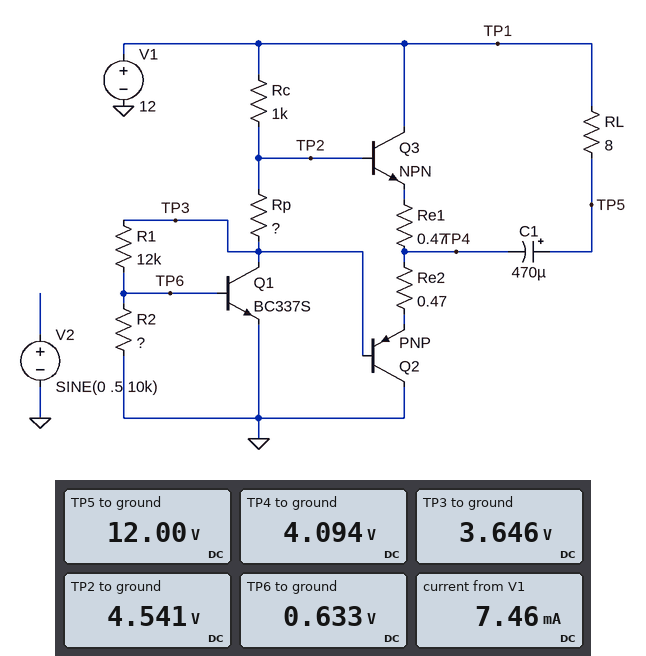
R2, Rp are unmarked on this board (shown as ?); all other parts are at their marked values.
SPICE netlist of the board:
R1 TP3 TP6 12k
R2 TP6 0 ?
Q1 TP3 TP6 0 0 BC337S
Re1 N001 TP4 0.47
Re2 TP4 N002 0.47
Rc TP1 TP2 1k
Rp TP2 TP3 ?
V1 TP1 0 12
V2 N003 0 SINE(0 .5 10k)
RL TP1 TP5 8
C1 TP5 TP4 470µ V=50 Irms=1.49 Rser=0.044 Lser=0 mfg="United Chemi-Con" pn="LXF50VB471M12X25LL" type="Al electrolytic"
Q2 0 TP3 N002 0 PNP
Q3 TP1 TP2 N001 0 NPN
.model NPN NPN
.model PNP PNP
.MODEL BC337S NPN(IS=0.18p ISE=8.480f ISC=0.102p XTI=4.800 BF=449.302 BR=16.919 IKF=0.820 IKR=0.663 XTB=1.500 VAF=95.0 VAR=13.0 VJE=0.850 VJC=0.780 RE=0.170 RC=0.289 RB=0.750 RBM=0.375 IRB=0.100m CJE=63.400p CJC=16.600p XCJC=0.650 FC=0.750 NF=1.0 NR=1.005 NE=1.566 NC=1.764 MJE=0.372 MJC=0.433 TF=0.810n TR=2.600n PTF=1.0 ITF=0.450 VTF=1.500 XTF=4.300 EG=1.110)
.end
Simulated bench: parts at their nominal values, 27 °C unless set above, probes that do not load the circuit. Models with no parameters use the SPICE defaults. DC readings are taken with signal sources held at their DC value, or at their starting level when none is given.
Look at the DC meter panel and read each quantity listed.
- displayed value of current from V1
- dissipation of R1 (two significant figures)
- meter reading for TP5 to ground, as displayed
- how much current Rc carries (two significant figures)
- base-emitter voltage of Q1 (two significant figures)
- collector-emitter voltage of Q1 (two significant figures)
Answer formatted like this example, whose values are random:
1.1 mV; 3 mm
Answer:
7.46 mA; 760 µW; 12.00 V; 7.5 mA; 630 mV; 3.6 V
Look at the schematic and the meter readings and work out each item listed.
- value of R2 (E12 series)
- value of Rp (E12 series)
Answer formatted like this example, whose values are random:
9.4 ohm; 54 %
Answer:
2.7 kΩ; 120 Ω
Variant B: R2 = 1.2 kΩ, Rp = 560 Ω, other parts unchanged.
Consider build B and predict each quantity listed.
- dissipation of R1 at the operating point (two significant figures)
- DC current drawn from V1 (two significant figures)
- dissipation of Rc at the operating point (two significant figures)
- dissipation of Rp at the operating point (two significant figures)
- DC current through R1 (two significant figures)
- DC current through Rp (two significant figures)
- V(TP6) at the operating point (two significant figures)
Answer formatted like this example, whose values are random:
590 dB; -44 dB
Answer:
3.2 mW; 36 mA; 12 mW; 5.5 mW; 510 µA; 3.1 mA; 610 mV
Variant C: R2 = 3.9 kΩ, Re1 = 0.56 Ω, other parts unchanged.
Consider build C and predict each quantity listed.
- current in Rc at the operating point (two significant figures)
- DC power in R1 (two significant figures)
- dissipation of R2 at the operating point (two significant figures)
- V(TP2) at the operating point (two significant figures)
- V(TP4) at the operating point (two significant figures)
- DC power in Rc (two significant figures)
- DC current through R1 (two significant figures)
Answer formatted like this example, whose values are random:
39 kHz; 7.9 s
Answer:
8.2 mA; 400 µW; 100 µW; 3.8 V; 3.3 V; 67 mW; 180 µA
